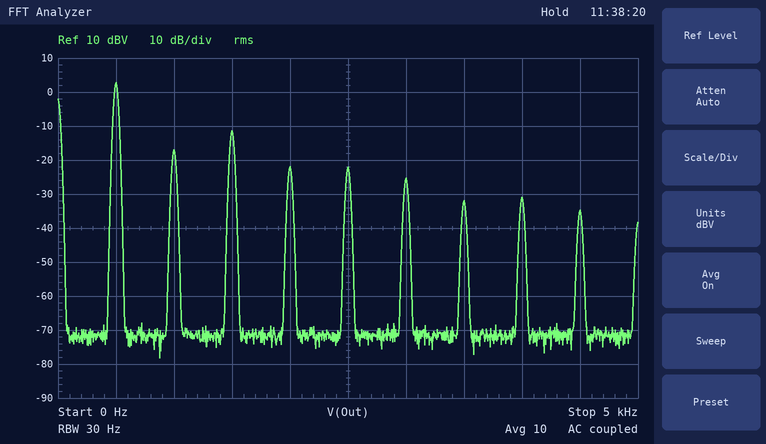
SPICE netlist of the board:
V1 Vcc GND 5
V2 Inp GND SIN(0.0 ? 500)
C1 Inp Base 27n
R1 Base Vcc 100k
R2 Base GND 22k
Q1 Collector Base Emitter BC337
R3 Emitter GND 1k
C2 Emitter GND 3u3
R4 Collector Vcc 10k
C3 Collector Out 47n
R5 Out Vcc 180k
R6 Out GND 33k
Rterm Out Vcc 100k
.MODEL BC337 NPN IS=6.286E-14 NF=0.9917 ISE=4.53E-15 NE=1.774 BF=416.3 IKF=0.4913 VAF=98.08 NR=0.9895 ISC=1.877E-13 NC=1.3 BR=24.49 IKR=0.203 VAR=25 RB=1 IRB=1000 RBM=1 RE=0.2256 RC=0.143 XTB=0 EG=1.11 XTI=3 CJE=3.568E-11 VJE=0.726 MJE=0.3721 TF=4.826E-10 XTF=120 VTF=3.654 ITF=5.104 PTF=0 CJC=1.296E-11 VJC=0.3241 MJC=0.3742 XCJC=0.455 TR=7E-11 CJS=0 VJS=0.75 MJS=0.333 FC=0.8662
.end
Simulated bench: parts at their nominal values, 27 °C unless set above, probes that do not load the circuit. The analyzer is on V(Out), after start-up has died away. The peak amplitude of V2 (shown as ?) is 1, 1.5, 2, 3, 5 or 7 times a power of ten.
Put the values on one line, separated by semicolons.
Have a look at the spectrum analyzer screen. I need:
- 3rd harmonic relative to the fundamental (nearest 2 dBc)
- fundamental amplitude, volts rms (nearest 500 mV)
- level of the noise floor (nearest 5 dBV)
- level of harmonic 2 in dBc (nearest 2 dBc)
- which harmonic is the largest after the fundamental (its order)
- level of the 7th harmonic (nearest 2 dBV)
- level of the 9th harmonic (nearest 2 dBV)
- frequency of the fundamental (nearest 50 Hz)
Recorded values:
-14 dBc; 1.5 V; -70 dBV; -20 dBc; 3; -32 dBV; -34 dBV; 500 Hz
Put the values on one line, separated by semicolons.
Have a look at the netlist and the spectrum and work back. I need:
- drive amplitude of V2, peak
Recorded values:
100 mV
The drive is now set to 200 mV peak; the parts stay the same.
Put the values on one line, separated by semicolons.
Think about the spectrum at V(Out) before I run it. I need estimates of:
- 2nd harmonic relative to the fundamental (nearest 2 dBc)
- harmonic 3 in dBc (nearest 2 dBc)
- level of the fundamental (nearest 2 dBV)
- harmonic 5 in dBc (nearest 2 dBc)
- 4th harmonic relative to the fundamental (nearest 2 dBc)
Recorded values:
-22 dBc; -12 dBc; 4 dBV; -20 dBc; -22 dBc
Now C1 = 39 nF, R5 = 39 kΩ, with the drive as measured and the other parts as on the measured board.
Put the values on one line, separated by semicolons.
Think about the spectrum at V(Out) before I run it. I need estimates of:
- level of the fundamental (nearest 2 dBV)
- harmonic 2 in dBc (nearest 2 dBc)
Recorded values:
2 dBV; -18 dBc
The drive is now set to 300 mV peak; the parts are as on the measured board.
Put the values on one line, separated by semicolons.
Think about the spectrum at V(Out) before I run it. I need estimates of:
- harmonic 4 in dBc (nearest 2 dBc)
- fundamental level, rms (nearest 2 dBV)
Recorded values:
-18 dBc; 4 dBV
